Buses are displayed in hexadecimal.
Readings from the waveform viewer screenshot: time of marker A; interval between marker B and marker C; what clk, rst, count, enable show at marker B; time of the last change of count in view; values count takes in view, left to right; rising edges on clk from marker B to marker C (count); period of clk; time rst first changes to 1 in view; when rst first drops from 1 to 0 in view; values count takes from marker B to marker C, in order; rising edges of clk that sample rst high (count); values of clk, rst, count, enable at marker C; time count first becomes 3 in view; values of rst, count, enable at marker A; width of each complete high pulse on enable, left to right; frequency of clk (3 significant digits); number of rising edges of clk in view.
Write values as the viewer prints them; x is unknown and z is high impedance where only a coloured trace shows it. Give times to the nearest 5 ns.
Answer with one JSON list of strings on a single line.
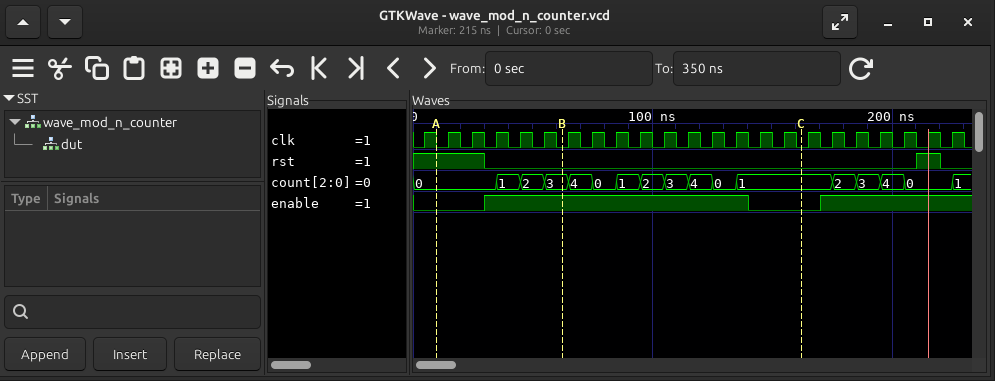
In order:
["10 ns", "100 ns", "clk=0, rst=0, count=3, enable=1", "225 ns", "0, 1, 2, 3, 4, 0, 1, 2, 3, 4, 0, 1, 2, 3, 4, 0, 1", "10", "10 ns", "210 ns", "30 ns", "3, 4, 0, 1, 2, 3, 4, 0, 1", "4", "clk=0, rst=0, count=1, enable=0", "55 ns", "rst=1, count=0, enable=0", "110 ns", "100 MHz", "23"]
